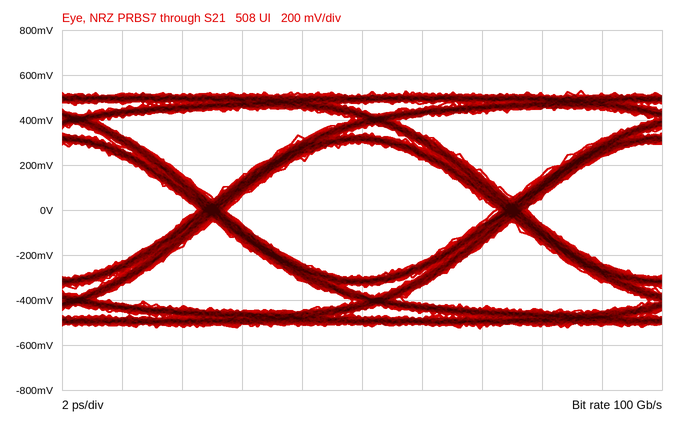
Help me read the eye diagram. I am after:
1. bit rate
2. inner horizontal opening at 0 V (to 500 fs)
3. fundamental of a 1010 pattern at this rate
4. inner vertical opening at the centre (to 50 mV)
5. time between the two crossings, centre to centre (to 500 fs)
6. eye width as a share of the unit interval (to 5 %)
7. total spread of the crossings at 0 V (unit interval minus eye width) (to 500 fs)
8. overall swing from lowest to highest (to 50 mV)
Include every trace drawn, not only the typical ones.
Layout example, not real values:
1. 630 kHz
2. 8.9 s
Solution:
1. 100 Gb/s
2. 9.0 ps
3. 50 GHz
4. 600 mV
5. 10.0 ps
6. 90 %
7. 1.0 ps
8. 1.05 V
